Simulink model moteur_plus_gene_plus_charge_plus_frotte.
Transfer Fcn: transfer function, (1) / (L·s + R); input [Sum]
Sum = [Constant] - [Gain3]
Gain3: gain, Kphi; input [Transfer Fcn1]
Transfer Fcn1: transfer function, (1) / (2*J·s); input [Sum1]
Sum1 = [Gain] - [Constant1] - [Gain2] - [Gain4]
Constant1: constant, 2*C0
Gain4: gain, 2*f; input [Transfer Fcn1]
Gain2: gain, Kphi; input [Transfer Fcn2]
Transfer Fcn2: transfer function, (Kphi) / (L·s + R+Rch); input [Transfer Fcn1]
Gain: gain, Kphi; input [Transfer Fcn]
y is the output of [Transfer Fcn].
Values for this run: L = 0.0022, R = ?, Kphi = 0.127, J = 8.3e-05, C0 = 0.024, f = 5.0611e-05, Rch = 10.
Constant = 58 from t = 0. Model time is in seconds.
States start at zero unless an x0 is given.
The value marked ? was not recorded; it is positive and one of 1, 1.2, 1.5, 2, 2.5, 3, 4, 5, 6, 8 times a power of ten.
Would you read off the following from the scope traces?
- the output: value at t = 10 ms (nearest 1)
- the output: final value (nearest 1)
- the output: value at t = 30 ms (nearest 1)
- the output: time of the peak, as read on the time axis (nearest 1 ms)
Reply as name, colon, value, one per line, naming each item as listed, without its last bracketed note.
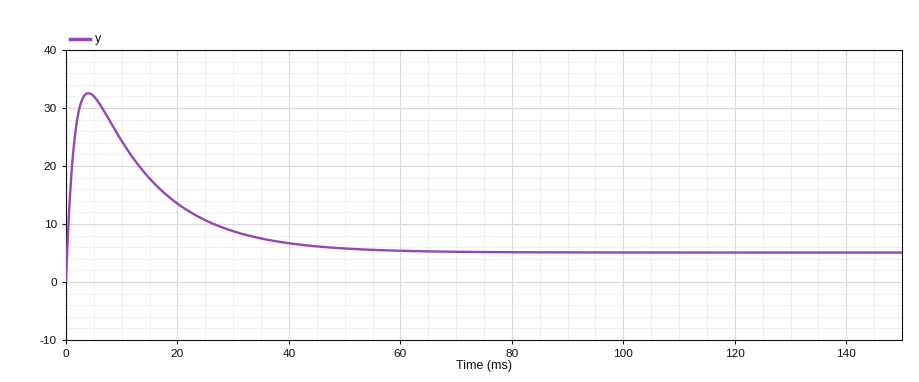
the output: value at t = 10 ms: 24
the output: final value: 5
the output: value at t = 30 ms: 9
the output: time of the peak, as read on the time axis: 4 ms
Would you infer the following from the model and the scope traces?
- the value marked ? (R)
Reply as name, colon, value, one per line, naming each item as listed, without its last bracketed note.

the value marked ?: 1.5
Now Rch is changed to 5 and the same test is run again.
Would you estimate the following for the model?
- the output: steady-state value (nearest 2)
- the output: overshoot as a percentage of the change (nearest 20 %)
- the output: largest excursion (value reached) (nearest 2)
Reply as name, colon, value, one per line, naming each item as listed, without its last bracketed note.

the output: steady-state value: 8
the output: overshoot as a percentage of the change: 320 %
the output: largest excursion (value reached): 32
